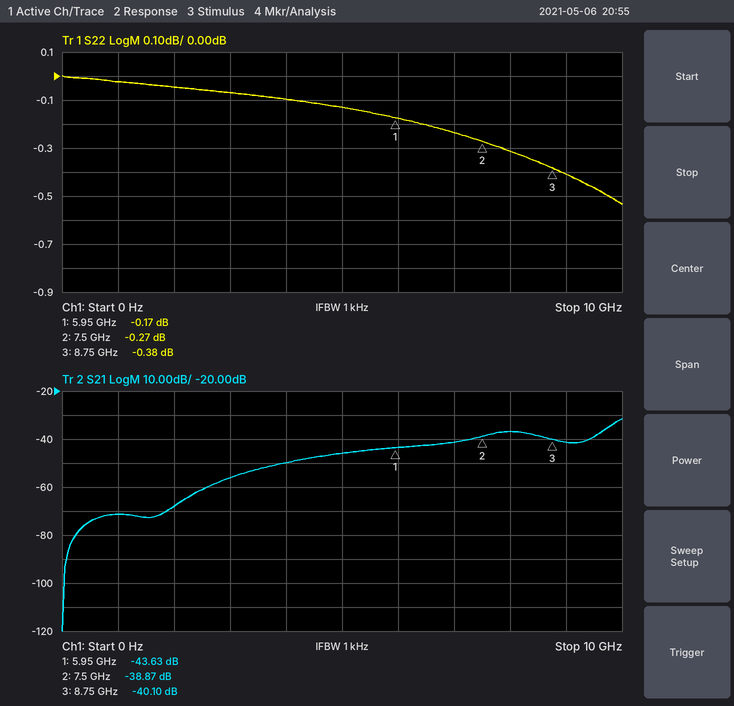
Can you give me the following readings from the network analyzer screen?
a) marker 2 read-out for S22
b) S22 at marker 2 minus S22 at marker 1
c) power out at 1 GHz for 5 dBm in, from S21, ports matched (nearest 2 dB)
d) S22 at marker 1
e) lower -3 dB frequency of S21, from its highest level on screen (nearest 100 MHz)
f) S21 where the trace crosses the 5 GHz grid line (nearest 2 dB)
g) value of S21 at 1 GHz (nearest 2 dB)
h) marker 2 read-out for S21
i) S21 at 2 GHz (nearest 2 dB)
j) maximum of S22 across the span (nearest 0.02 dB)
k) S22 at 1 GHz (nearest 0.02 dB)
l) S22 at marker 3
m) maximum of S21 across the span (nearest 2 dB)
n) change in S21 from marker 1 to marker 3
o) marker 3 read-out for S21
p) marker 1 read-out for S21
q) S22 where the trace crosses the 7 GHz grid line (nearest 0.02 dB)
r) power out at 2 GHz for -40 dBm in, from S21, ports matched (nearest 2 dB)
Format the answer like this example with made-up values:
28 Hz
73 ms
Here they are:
-0.27 dB
-0.10 dB
-66 dBm
-0.17 dB
9.8 GHz
-46 dB
-72 dB
-38.87 dB
-68 dB
0.00 dB
-0.02 dB
-0.38 dB
-32 dB
3.53 dB
-40.10 dB
-43.63 dB
-0.24 dB
-108 dBm
